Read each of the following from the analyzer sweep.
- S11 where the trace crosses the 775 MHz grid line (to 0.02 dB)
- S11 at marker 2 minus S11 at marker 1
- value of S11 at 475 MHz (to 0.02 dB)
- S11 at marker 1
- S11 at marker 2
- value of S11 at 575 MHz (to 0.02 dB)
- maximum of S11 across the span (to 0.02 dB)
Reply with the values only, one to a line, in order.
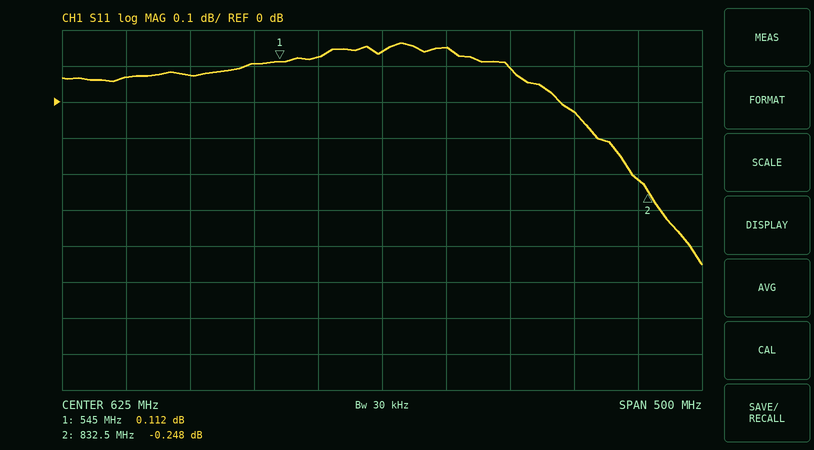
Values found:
-0.02 dB
-0.360 dB
0.08 dB
0.112 dB
-0.248 dB
0.12 dB
0.16 dB
